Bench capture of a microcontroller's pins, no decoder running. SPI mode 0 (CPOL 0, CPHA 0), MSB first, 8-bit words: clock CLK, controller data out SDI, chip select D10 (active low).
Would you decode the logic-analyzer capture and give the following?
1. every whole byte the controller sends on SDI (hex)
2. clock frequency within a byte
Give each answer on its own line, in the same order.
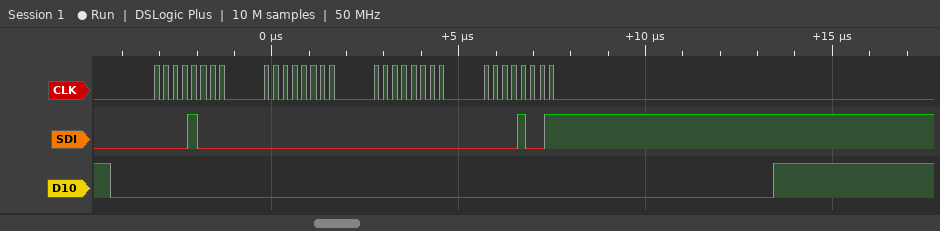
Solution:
08 00 00 09
4 MHz
